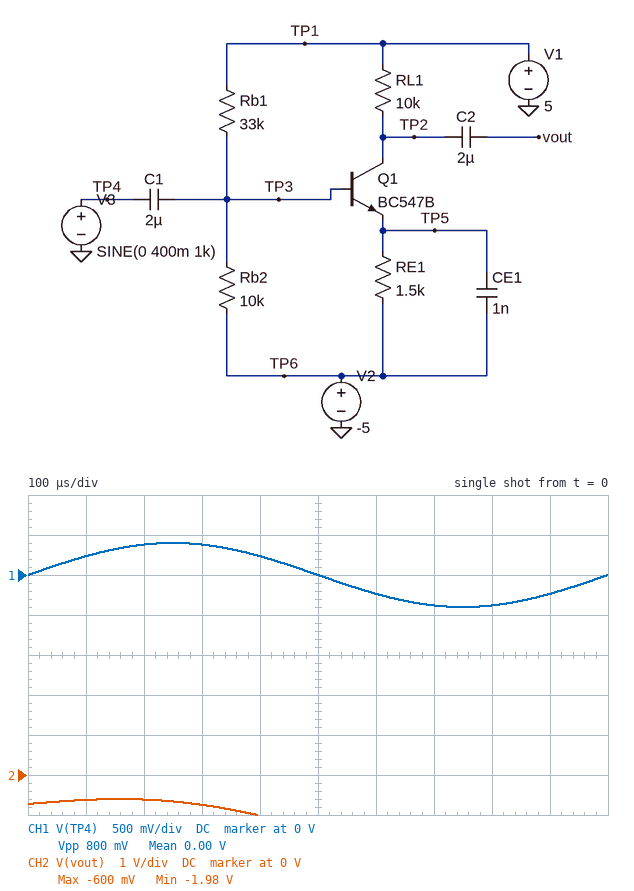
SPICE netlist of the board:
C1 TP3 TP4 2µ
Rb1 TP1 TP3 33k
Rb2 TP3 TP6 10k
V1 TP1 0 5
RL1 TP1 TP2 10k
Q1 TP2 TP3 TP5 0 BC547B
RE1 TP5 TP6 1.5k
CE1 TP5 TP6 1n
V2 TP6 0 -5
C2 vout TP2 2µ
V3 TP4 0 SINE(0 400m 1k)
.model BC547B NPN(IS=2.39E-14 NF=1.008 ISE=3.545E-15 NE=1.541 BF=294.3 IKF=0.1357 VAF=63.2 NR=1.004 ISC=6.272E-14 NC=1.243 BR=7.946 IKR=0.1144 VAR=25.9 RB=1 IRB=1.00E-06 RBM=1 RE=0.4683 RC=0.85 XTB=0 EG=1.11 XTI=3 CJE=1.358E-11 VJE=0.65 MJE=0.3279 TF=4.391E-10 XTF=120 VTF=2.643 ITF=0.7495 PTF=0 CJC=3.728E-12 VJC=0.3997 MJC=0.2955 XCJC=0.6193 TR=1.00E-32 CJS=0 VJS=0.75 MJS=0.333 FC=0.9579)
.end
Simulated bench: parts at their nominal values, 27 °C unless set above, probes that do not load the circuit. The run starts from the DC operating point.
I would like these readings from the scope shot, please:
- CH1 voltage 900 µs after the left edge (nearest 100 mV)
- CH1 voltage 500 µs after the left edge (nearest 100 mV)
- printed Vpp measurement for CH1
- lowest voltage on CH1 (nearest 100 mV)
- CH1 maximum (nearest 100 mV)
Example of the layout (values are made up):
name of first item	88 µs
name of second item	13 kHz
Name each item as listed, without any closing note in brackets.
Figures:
CH1 voltage 900 µs after the left edge	-200 mV
CH1 voltage 500 µs after the left edge	0 V
printed Vpp measurement for CH1	800 mV
lowest voltage on CH1	-400 mV
CH1 maximum	400 mV
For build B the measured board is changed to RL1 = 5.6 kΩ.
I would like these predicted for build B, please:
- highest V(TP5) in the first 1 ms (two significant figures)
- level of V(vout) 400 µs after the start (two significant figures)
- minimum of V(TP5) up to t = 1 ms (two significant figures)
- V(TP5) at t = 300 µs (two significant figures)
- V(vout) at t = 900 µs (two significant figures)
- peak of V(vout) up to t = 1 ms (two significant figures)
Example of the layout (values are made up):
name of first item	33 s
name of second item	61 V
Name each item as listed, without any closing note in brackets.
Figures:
highest V(TP5) in the first 1 ms	-570 mV
level of V(vout) 400 µs after the start	-920 mV
minimum of V(TP5) up to t = 1 ms	-1.8 V
V(TP5) at t = 300 µs	-690 mV
V(vout) at t = 900 µs	-1.7 V
peak of V(vout) up to t = 1 ms	-560 mV
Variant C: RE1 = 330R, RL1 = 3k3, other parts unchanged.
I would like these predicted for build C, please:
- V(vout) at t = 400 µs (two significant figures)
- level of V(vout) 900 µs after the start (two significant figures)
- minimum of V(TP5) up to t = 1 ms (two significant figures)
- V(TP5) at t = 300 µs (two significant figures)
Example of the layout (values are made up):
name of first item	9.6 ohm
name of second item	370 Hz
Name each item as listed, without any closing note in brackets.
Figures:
V(vout) at t = 400 µs	-2.3 V
level of V(vout) 900 µs after the start	-3.5 V
minimum of V(TP5) up to t = 1 ms	-3.6 V
V(TP5) at t = 300 µs	-1.9 V
